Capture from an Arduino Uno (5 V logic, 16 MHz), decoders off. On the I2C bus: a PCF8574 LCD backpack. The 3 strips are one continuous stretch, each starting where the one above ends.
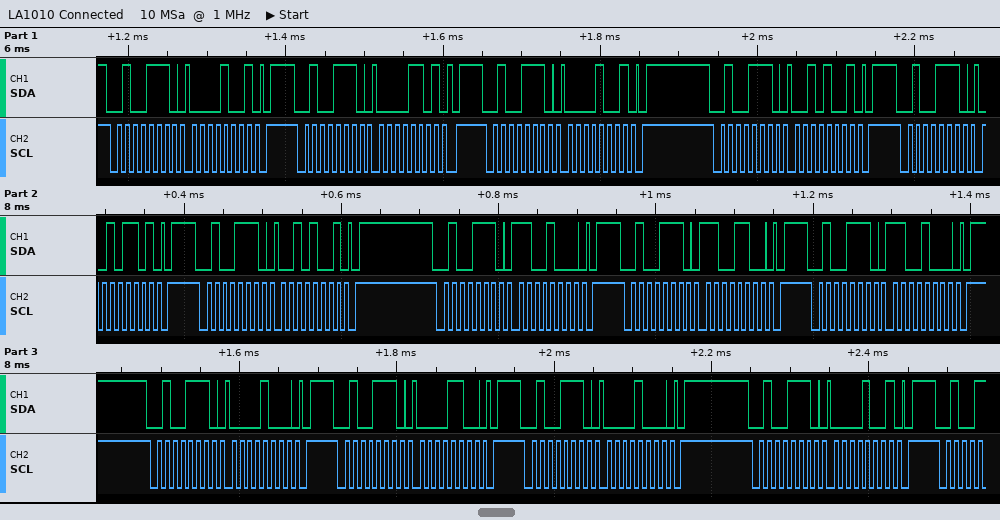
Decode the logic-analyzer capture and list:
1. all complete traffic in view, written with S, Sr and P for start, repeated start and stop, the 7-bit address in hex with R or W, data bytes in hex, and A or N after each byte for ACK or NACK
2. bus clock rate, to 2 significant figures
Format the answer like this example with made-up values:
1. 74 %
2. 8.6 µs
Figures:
1. S 27W A 09 A P S 27W A 0D A P S 27W A 09 A P S 27W A 29 A P S 27W A 2D A P S 27W A 29 A P S 27W A C8 A P S 27W A CC A P S 27W A C8 A P S 27W A 08 A P S 27W A 0C A P S 27W A 08 A P S 27W A 09 A P
2. 100 kHz
